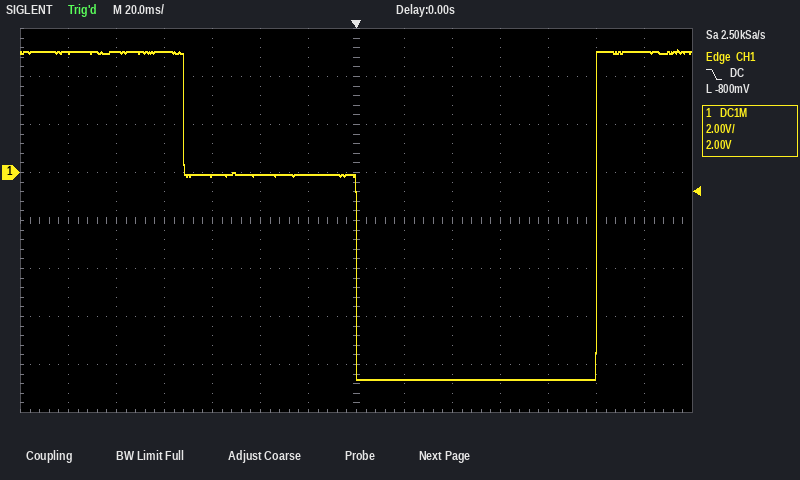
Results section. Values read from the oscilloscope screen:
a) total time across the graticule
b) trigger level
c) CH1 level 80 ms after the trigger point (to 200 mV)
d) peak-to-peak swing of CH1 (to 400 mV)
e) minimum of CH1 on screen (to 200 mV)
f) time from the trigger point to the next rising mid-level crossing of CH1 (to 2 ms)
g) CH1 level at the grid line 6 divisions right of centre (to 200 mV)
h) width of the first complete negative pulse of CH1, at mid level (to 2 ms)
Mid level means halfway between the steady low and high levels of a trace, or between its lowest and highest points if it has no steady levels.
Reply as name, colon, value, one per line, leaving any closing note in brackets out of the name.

total time across the graticule: 280 ms
trigger level: -800 mV
CH1 level 80 ms after the trigger point: -8.6 V
peak-to-peak swing of CH1: 13.6 V
minimum of CH1 on screen: -8.6 V
time from the trigger point to the next rising mid-level crossing of CH1: 100 ms
CH1 level at the grid line 6 divisions right of centre: 5.0 V
width of the first complete negative pulse of CH1, at mid level: 100 ms
